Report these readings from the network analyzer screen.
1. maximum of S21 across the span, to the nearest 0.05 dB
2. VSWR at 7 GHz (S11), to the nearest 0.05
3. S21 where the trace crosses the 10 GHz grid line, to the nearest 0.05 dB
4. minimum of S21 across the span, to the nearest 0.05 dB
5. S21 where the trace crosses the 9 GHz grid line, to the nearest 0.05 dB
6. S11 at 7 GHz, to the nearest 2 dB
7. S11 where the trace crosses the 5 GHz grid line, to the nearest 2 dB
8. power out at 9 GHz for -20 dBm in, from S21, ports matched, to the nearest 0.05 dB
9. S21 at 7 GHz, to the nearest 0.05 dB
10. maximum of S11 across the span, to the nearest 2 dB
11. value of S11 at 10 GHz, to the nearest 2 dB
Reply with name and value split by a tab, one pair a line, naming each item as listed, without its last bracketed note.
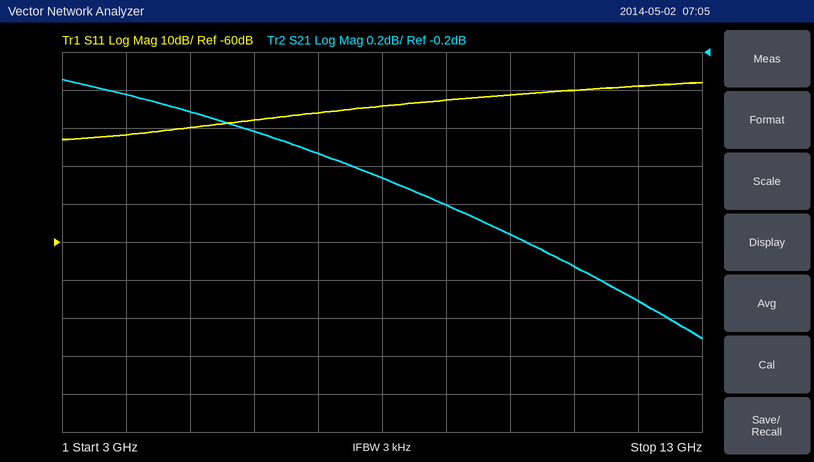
maximum of S21 across the span, to the nearest 0.05 dB	-0.35 dB
VSWR at 7 GHz (S11), to the nearest 0.05	1.10
S21 where the trace crosses the 10 GHz grid line, to the nearest 0.05 dB	-1.15 dB
minimum of S21 across the span, to the nearest 0.05 dB	-1.70 dB
S21 where the trace crosses the 9 GHz grid line, to the nearest 0.05 dB	-1.00 dB
S11 at 7 GHz, to the nearest 2 dB	-26 dB
S11 where the trace crosses the 5 GHz grid line, to the nearest 2 dB	-30 dB
power out at 9 GHz for -20 dBm in, from S21, ports matched, to the nearest 0.05 dB	-21.00 dBm
S21 at 7 GHz, to the nearest 0.05 dB	-0.75 dB
maximum of S11 across the span, to the nearest 2 dB	-18 dB
value of S11 at 10 GHz, to the nearest 2 dB	-22 dB
